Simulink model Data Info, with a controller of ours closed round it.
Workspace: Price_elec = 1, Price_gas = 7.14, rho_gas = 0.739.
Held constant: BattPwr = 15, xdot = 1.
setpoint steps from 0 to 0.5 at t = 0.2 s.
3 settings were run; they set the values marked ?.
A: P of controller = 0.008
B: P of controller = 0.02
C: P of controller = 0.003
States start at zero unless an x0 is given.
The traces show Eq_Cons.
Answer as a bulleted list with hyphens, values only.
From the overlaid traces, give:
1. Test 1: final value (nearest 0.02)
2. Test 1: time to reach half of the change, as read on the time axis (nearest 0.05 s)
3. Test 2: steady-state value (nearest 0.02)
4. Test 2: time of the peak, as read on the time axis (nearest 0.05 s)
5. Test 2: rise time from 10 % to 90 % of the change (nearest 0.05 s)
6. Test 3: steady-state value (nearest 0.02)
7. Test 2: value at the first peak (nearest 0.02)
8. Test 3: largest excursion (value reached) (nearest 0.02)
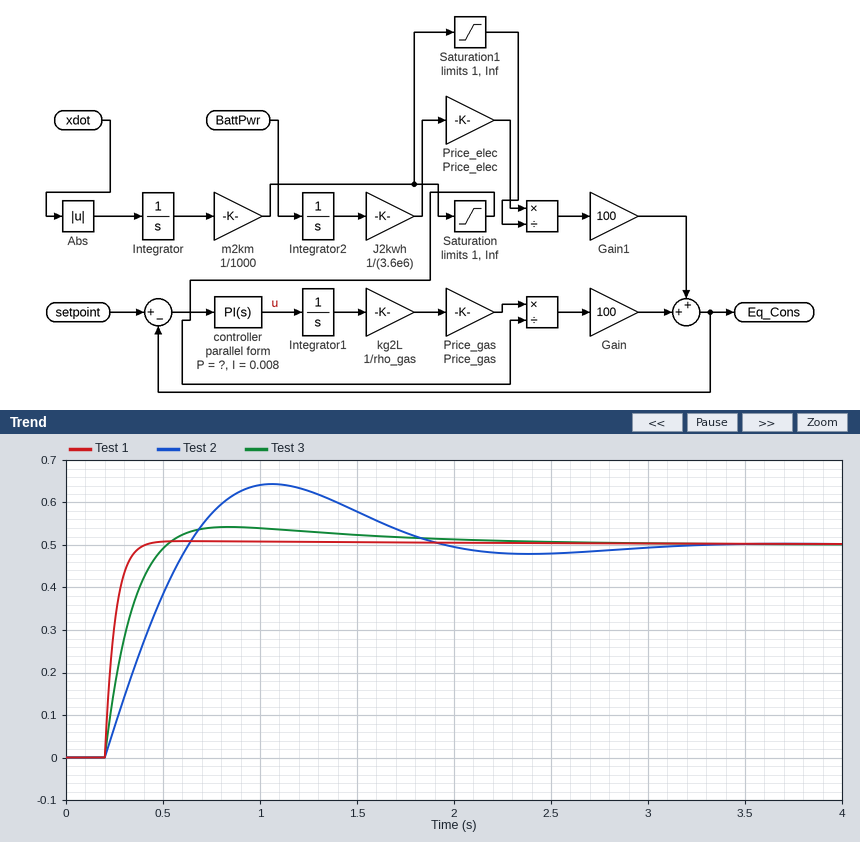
- 0.50
- 0.25 s
- 0.50
- 1.05 s
- 0.35 s
- 0.50
- 0.64
- 0.54
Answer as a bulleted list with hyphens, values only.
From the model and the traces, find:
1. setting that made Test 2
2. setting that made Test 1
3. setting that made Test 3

- C
- B
- A
